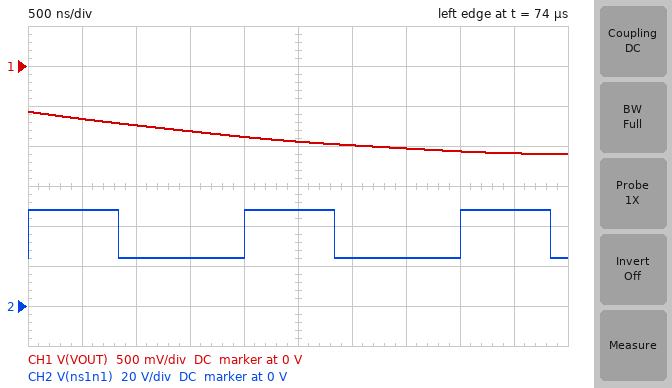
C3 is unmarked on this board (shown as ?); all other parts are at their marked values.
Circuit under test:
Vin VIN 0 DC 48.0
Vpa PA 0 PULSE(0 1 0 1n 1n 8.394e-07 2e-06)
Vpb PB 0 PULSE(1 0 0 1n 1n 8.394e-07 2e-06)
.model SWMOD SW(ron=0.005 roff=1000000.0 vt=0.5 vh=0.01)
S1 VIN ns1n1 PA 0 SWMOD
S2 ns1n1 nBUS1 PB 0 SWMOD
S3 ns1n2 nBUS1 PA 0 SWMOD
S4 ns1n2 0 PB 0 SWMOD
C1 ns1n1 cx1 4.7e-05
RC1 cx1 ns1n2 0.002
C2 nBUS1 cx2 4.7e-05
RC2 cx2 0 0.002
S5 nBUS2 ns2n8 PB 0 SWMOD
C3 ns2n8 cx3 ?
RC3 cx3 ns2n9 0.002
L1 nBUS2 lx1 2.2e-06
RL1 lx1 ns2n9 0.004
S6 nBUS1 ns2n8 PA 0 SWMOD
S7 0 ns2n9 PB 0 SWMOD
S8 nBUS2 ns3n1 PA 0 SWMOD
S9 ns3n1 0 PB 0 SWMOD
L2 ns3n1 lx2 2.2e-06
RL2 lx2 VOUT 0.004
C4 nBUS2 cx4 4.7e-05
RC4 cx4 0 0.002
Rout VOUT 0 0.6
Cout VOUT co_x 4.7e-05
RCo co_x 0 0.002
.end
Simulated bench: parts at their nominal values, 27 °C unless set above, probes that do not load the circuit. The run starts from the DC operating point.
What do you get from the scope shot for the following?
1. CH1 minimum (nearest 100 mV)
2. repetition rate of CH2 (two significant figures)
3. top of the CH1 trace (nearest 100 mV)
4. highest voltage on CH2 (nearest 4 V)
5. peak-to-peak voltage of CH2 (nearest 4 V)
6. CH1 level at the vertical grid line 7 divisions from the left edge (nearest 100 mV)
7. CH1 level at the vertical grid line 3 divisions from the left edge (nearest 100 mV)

-1.1 V
500 kHz
-600 mV
48 V
24 V
-1.0 V
-800 mV
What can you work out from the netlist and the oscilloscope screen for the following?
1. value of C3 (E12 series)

56 µF
